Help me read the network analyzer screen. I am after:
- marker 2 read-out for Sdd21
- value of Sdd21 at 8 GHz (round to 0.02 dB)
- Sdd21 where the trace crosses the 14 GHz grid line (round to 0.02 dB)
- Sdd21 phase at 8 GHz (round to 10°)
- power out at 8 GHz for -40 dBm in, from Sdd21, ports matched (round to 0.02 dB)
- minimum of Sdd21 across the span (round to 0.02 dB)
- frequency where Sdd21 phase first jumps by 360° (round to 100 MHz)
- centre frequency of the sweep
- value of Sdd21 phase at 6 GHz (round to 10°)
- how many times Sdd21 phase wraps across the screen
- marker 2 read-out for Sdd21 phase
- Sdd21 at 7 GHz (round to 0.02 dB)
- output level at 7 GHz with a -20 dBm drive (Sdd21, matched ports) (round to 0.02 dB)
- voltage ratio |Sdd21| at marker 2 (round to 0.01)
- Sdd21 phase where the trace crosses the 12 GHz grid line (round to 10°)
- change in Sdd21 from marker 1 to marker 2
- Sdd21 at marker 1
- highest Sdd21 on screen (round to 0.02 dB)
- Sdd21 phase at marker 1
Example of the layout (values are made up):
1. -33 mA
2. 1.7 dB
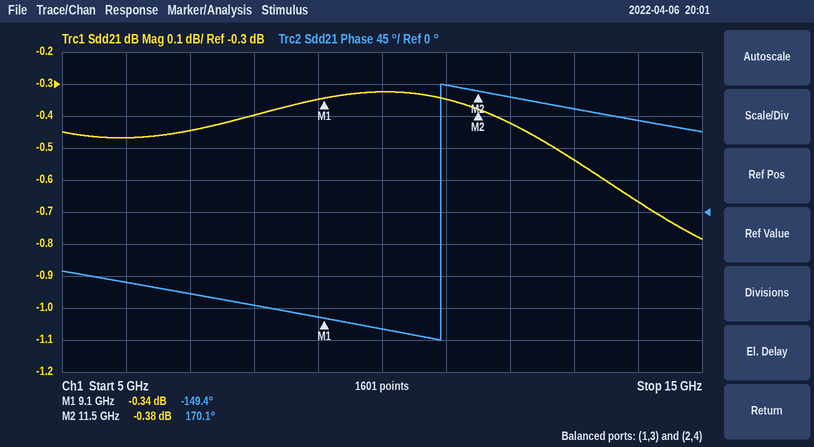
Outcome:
1. -0.38 dB
2. -0.40 dB
3. -0.66 dB
4. -130°
5. -40.40 dBm
6. -0.78 dB
7. 10.9 GHz
8. 10 GHz
9. -100°
10. 1
11. 170.1°
12. -0.44 dB
13. -20.44 dBm
14. 0.96
15. 160°
16. -0.04 dB
17. -0.34 dB
18. -0.32 dB
19. -149.4°
